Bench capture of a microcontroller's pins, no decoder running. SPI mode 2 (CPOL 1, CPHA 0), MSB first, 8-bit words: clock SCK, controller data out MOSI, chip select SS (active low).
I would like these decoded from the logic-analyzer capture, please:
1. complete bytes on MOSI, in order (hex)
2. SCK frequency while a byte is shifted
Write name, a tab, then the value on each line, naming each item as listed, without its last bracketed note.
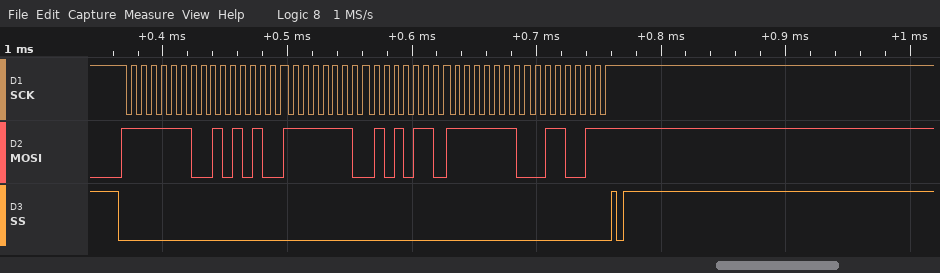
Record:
complete bytes on MOSI, in order	FE 54 FE 56 FE 33
SCK frequency while a byte is shifted	125 kHz
